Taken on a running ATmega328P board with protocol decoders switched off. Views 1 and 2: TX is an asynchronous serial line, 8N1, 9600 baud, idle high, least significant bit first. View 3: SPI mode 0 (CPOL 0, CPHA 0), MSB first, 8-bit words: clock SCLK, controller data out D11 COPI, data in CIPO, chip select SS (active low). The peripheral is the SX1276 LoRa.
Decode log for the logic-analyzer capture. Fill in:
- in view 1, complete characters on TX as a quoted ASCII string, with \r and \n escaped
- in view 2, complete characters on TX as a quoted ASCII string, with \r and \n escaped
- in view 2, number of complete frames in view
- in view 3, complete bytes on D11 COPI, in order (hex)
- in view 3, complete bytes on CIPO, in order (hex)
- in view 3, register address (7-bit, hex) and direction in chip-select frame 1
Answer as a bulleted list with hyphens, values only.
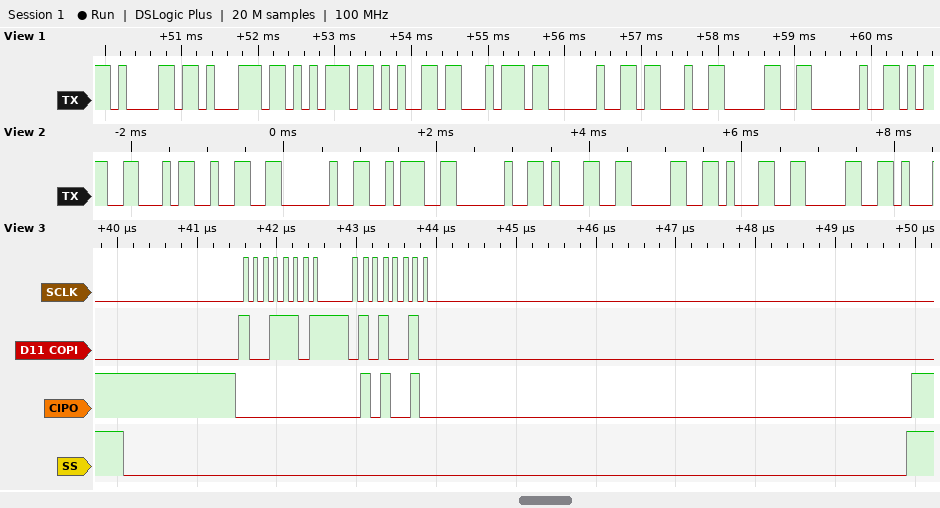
- "aquet #0 "
- "F2 : 1010"
- 9
- 9D 52
- 00 52
- 0x1D write
